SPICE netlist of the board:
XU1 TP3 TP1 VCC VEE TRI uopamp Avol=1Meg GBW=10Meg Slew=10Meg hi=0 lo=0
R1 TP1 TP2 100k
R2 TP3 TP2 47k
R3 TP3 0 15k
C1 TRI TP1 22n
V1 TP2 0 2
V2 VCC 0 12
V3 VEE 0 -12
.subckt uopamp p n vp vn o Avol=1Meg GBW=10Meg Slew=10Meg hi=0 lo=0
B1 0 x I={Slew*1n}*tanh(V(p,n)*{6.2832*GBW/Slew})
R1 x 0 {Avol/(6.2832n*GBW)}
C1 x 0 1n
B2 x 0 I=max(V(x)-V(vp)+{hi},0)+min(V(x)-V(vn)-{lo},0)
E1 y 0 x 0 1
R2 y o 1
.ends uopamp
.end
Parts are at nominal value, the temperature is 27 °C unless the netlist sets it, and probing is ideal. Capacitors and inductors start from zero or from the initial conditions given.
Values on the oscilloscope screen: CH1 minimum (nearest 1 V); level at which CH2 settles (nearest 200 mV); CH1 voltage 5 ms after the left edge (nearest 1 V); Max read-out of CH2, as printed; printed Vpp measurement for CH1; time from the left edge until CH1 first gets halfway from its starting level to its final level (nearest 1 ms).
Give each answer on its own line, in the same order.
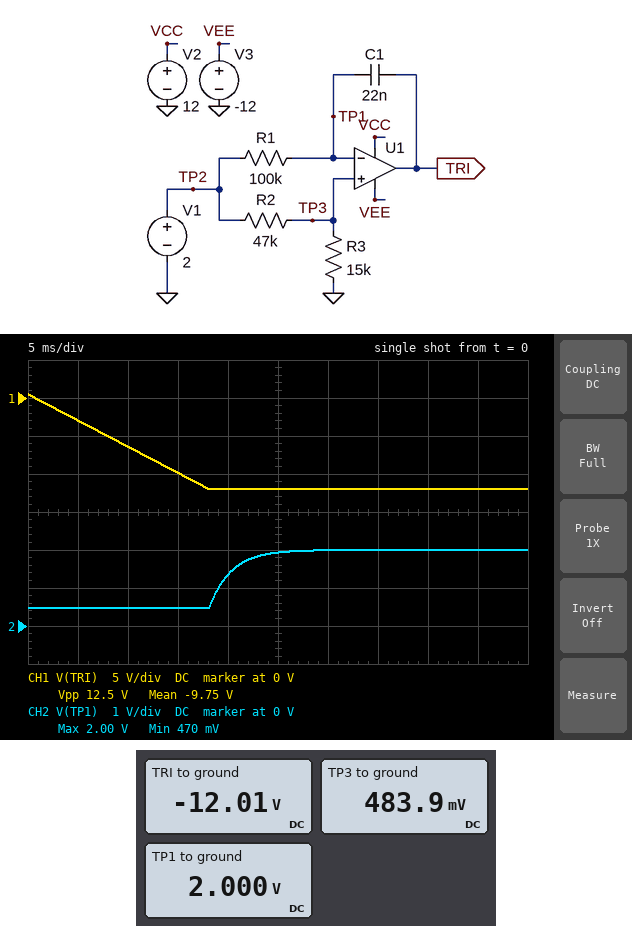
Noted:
-12 V
2.0 V
-3 V
2.00 V
12.5 V
9 ms
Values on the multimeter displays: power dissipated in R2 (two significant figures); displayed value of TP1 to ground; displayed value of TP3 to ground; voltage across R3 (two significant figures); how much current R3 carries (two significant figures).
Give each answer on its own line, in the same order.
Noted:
49 µW
2.000 V
483.9 mV
480 mV
32 µA
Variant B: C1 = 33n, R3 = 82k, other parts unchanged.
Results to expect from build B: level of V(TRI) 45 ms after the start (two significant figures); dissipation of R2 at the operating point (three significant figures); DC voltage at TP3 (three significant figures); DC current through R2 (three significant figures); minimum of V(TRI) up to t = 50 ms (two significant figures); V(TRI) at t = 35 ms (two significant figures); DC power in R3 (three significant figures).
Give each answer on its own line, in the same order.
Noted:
-8.7 V
11.3 µW
1.27 V
15.5 µA
-9.8 V
-6.5 V
19.7 µW
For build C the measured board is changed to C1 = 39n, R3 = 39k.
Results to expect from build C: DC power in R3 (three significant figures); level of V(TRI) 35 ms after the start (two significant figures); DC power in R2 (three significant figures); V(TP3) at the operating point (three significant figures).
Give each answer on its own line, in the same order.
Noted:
21.1 µW
-8.9 V
25.4 µW
907 mV
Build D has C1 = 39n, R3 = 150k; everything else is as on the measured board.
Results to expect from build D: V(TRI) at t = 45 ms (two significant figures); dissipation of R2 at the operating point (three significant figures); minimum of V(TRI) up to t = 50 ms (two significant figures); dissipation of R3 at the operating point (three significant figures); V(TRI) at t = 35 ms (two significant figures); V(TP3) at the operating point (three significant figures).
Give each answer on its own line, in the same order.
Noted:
-4.0 V
4.84 µW
-4.6 V
15.5 µW
-2.8 V
1.52 V
